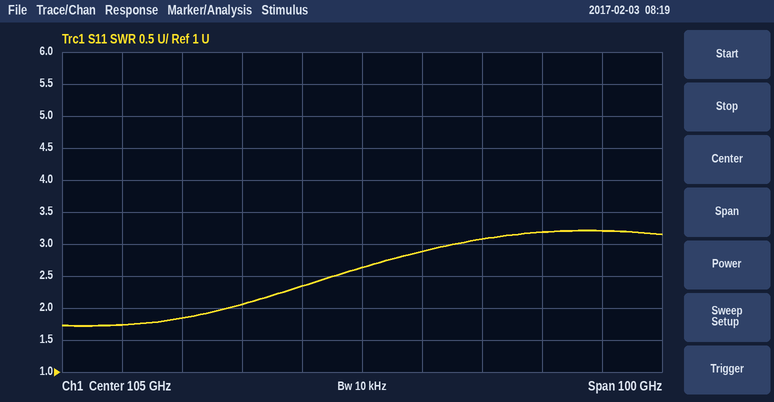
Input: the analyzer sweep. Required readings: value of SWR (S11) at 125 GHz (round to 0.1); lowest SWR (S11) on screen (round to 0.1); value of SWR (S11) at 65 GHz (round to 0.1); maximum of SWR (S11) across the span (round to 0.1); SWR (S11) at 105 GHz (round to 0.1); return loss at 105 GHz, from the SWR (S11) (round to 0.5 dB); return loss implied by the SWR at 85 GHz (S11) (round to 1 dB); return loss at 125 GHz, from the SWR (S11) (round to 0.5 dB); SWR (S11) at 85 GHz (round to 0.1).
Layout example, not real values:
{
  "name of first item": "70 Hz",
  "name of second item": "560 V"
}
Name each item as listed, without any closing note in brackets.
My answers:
{
  "value of SWR (S11) at 125 GHz": "3.1",
  "lowest SWR (S11) on screen": "1.7",
  "value of SWR (S11) at 65 GHz": "1.7",
  "maximum of SWR (S11) across the span": "3.2",
  "SWR (S11) at 105 GHz": "2.6",
  "return loss at 105 GHz, from the SWR (S11)": "7.0 dB",
  "return loss implied by the SWR at 85 GHz (S11)": "9 dB",
  "return loss at 125 GHz, from the SWR (S11)": "6.0 dB",
  "SWR (S11) at 85 GHz": "2.1"
}
